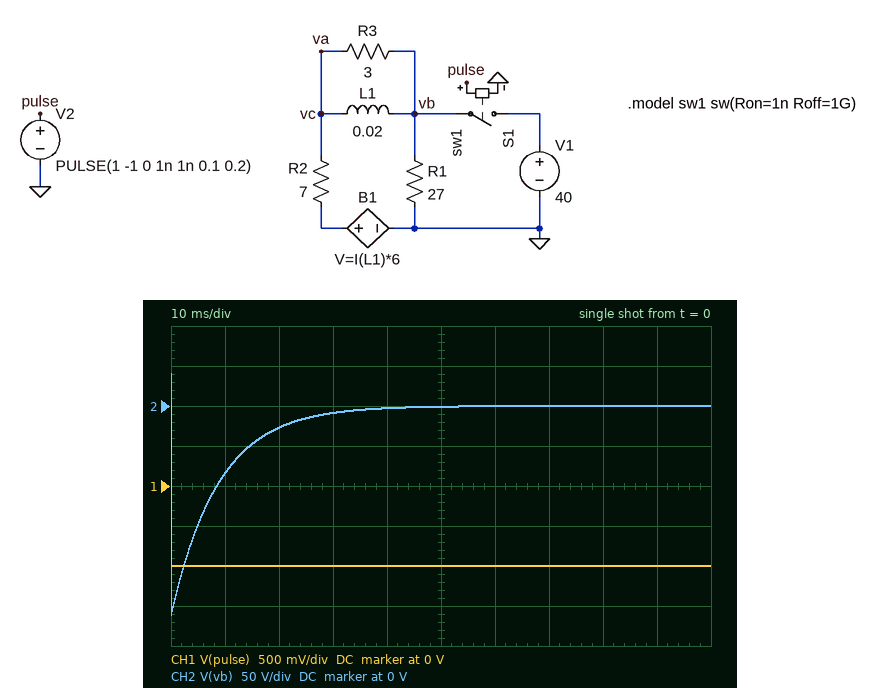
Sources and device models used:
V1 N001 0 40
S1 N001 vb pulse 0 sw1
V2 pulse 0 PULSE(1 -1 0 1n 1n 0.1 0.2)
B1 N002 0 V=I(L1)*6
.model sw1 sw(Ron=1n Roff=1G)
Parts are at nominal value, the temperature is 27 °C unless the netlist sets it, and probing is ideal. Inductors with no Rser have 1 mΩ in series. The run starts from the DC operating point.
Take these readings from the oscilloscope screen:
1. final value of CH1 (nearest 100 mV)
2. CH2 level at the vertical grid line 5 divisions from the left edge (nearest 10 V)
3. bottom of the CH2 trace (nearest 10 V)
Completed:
-1.0 V
0 V
-260 V
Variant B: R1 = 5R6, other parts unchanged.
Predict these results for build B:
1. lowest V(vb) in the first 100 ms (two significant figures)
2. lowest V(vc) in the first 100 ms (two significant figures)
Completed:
-130 V
-78 V
